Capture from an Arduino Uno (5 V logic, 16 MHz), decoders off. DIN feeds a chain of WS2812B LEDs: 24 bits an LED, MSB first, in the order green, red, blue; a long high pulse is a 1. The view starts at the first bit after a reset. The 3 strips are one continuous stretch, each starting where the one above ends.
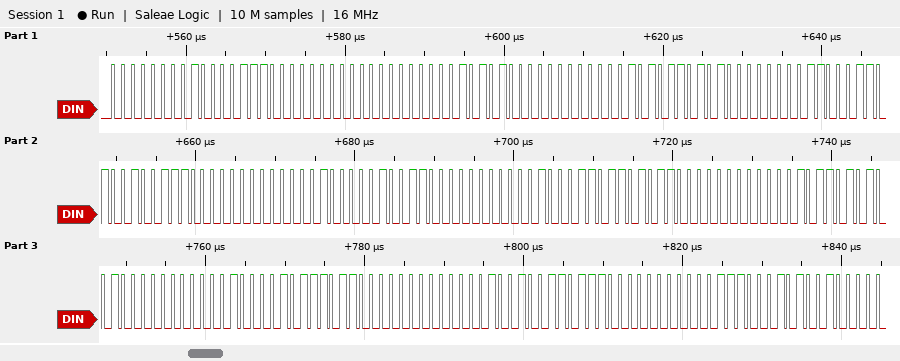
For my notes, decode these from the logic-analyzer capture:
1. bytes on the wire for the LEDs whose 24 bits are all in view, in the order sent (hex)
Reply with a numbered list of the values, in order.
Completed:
1. 00 87 00 00 15 00 0A D4 03 1A 4E 00 08 26 00 23 6B 00 0B 52 00 21 76 00 09 37 00
